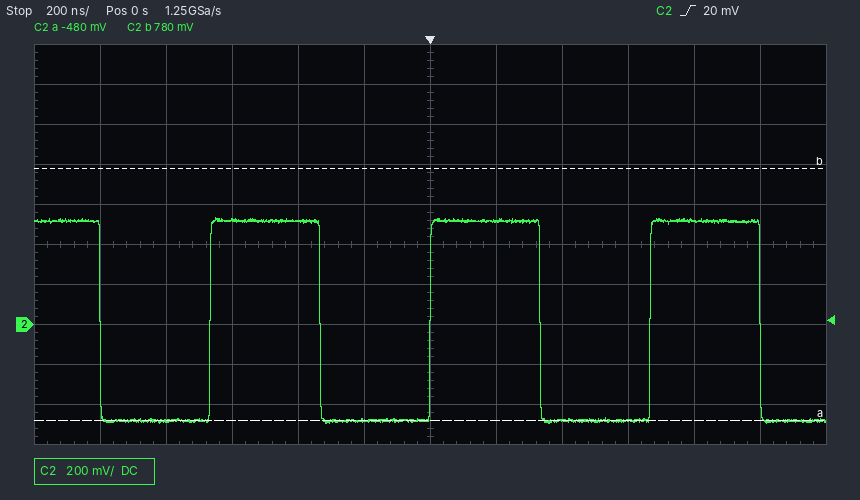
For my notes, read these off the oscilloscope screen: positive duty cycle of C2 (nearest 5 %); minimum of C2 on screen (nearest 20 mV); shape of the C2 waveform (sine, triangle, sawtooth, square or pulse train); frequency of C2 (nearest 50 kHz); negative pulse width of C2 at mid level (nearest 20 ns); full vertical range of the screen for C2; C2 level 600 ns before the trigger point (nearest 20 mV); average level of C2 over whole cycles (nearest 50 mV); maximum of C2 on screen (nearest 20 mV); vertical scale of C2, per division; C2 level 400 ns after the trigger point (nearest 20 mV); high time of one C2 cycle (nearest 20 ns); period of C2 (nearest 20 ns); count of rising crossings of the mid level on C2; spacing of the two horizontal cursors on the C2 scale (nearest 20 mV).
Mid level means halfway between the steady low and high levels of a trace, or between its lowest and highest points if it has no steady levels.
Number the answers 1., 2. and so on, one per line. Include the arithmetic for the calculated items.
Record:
1. 340 ns / 660 ns ≈ 51.5 %, so 50 % to the nearest 5 %
2. -500 mV
3. square
4. 1 / 660 ns ≈ 1.52 MHz, so 1.50 MHz to the nearest 50 kHz
5. 340 ns
6. 2 V
7. 520 mV
8. -500 mV + 0.5 × (540 mV − (-500 mV)) ≈ 0 mV
9. 540 mV
10. 200 mV
11. -480 mV
12. 340 ns
13. 660 ns
14. 3
15. 1.26 V
